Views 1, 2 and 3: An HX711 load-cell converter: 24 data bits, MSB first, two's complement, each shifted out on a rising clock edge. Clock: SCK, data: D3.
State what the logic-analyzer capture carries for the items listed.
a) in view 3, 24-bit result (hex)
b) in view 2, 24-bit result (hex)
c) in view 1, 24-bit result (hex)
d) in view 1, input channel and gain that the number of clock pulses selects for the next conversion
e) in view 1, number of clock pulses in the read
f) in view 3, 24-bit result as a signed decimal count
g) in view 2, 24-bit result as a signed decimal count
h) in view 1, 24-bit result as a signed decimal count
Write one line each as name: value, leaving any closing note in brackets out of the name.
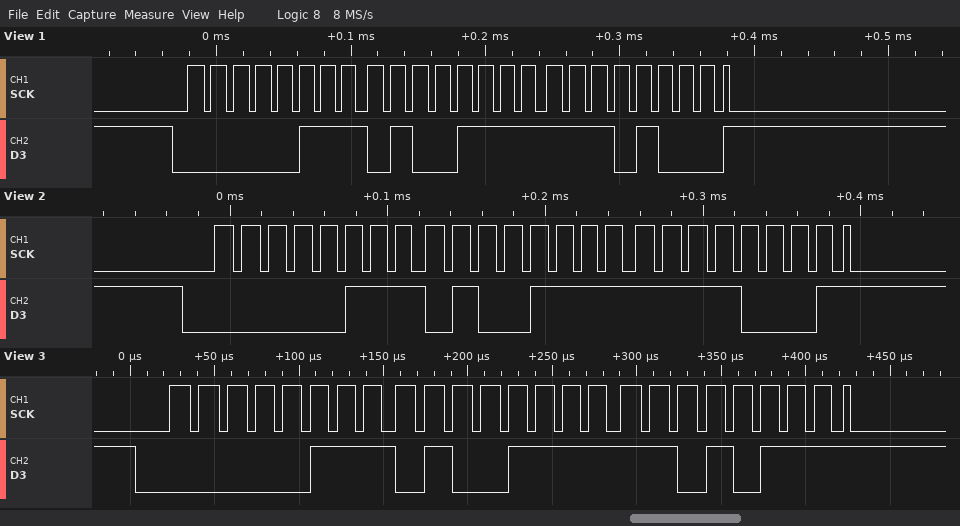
in view 3, 24-bit result: 0x074FD7
in view 2, 24-bit result: 0x074FF1
in view 1, 24-bit result: 0x074FE8
in view 1, input channel and gain that the number of clock pulses selects for the next conversion: channel A, gain 128
in view 1, number of clock pulses in the read: 25
in view 3, 24-bit result as a signed decimal count: 479191
in view 2, 24-bit result as a signed decimal count: 479217
in view 1, 24-bit result as a signed decimal count: 479208
